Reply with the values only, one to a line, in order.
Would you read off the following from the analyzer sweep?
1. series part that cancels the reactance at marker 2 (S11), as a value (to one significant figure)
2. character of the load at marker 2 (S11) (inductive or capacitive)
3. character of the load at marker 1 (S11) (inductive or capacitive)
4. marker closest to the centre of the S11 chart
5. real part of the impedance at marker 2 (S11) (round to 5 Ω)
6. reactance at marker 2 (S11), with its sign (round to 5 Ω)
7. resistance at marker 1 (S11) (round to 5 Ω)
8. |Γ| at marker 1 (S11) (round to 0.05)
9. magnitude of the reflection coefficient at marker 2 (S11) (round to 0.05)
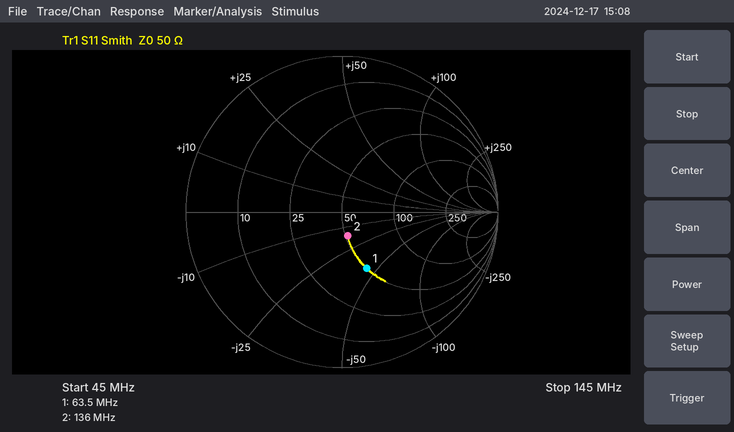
20 nH
capacitive
capacitive
marker 2
50 Ω
-15 Ω
50 Ω
0.40
0.15
